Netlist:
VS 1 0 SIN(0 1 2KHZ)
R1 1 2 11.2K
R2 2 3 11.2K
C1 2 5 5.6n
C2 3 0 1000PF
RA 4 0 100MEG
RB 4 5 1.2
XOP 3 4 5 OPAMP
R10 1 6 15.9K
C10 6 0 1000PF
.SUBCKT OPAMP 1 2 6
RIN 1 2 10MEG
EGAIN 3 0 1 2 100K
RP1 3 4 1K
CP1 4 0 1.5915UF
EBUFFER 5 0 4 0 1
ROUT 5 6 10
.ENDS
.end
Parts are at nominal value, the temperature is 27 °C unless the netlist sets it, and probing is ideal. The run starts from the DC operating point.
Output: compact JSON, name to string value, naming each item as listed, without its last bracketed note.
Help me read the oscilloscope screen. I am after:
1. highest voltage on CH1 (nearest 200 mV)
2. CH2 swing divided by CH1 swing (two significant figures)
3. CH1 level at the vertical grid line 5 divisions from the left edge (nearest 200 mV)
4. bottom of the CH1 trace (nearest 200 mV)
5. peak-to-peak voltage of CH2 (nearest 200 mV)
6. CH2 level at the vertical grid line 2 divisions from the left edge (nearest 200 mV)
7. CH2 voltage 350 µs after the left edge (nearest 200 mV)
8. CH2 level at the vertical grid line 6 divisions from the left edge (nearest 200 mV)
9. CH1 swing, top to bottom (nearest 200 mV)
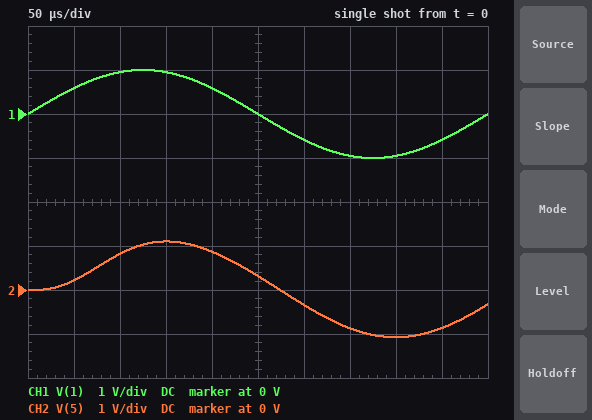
{"highest voltage on CH1": "1.0 V", "CH2 swing divided by CH1 swing": "1.1", "CH1 level at the vertical grid line 5 divisions from the left edge": "0 V", "bottom of the CH1 trace": "-1.0 V", "peak-to-peak voltage of CH2": "2.2 V", "CH2 level at the vertical grid line 2 divisions from the left edge": "800 mV", "CH2 voltage 350 µs after the left edge": "-800 mV", "CH2 level at the vertical grid line 6 divisions from the left edge": "-400 mV", "CH1 swing, top to bottom": "2.0 V"}
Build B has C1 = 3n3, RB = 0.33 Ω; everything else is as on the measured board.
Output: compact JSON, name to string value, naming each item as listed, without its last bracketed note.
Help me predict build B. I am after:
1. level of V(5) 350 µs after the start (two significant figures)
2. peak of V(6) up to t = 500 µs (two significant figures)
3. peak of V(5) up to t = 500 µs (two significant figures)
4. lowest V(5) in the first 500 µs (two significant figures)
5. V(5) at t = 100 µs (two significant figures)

{"level of V(5) 350 µs after the start": "-840 mV", "peak of V(6) up to t = 500 µs": "980 mV", "peak of V(5) up to t = 500 µs": "1.0 V", "lowest V(5) in the first 500 µs": "-1.0 V", "V(5) at t = 100 µs": "840 mV"}
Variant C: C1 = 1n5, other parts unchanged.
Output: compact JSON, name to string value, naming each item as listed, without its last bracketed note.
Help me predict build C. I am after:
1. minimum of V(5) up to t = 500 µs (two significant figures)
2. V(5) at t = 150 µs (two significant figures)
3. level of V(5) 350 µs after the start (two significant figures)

{"minimum of V(5) up to t = 500 µs": "-990 mV", "V(5) at t = 150 µs": "990 mV", "level of V(5) 350 µs after the start": "-820 mV"}
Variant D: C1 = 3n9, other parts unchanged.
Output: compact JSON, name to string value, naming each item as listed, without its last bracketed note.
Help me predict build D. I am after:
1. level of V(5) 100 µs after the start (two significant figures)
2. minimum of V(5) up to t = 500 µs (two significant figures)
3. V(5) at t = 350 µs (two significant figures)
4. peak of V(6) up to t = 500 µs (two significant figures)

{"level of V(5) 100 µs after the start": "840 mV", "minimum of V(5) up to t = 500 µs": "-1.0 V", "V(5) at t = 350 µs": "-850 mV", "peak of V(6) up to t = 500 µs": "980 mV"}
